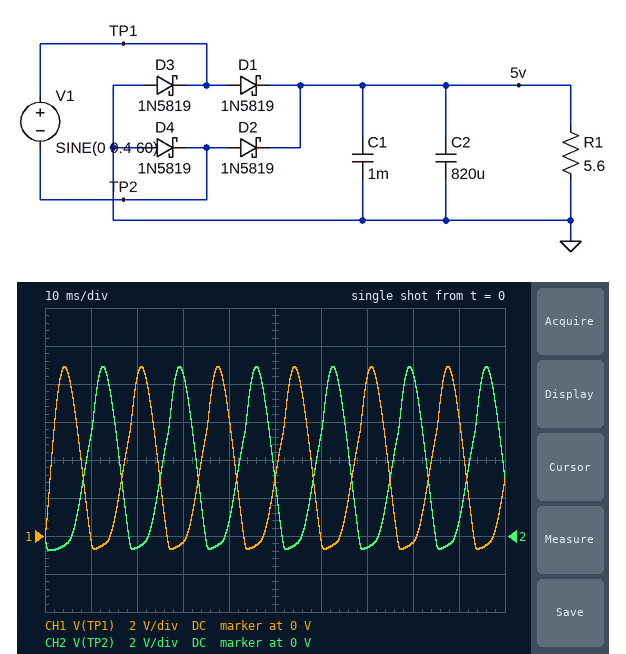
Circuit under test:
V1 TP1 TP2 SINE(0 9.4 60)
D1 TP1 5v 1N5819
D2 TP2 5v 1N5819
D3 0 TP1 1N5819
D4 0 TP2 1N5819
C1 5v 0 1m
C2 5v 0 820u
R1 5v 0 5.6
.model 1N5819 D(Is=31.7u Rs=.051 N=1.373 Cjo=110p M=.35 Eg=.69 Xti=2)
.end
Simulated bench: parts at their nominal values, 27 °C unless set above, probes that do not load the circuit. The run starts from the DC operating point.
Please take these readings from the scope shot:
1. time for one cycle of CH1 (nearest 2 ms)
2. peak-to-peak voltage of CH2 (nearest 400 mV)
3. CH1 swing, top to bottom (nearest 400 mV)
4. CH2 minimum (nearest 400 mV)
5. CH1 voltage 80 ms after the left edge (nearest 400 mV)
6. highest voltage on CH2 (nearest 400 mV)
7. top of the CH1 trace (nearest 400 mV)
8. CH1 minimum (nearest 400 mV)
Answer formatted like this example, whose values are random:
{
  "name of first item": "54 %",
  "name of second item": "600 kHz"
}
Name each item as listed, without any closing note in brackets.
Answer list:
{
  "time for one cycle of CH1": "16 ms",
  "peak-to-peak voltage of CH2": "9.6 V",
  "CH1 swing, top to bottom": "9.6 V",
  "CH2 minimum": "-800 mV",
  "CH1 voltage 80 ms after the left edge": "-400 mV",
  "highest voltage on CH2": "8.8 V",
  "top of the CH1 trace": "8.8 V",
  "CH1 minimum": "-800 mV"
}
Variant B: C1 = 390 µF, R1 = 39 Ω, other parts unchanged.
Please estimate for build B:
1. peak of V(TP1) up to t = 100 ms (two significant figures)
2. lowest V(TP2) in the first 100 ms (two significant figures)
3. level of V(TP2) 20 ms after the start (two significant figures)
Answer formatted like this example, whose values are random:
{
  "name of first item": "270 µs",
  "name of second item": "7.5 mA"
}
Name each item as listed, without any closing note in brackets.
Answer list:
{
  "peak of V(TP1) up to t = 100 ms": "9.0 V",
  "lowest V(TP2) in the first 100 ms": "-630 mV",
  "level of V(TP2) 20 ms after the start": "-470 mV"
}
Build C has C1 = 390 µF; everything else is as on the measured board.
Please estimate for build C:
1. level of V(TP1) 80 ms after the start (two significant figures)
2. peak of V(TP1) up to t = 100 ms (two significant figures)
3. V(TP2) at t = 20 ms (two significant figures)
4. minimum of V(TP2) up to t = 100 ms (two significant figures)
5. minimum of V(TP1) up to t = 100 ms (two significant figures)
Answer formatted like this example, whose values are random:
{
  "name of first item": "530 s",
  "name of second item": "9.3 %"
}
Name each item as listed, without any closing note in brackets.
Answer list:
{
  "level of V(TP1) 80 ms after the start": "-370 mV",
  "peak of V(TP1) up to t = 100 ms": "8.9 V",
  "V(TP2) at t = 20 ms": "-550 mV",
  "minimum of V(TP2) up to t = 100 ms": "-640 mV",
  "minimum of V(TP1) up to t = 100 ms": "-620 mV"
}
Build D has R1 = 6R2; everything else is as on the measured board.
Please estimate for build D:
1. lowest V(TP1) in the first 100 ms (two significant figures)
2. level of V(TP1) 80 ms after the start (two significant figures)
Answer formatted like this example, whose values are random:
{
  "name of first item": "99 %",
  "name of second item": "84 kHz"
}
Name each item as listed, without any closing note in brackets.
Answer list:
{
  "lowest V(TP1) in the first 100 ms": "-670 mV",
  "level of V(TP1) 80 ms after the start": "-330 mV"
}
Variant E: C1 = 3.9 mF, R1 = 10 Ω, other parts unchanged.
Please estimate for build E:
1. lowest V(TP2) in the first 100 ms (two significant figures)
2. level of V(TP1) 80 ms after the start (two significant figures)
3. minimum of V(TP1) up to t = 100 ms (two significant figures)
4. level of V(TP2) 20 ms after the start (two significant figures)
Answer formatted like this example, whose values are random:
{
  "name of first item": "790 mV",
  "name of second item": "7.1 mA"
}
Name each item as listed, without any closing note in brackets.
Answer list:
{
  "lowest V(TP2) in the first 100 ms": "-1.2 V",
  "level of V(TP1) 80 ms after the start": "-290 mV",
  "minimum of V(TP1) up to t = 100 ms": "-670 mV",
  "level of V(TP2) 20 ms after the start": "-660 mV"
}
